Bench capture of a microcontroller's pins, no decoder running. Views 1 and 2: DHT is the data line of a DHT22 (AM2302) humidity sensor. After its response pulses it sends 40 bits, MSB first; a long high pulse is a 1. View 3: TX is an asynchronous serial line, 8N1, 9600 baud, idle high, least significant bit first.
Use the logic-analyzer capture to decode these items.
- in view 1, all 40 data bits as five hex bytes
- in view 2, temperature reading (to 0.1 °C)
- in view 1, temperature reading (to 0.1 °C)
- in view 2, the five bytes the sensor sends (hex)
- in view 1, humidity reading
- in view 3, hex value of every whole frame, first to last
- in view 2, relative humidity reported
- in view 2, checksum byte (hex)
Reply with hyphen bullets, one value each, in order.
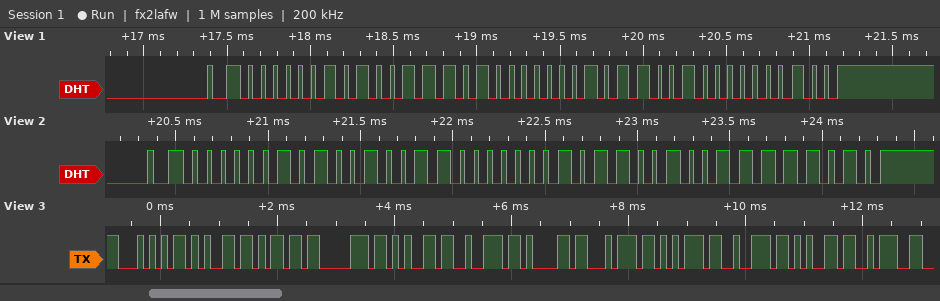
- 02 9D 01 64 04
- 35.6 °C
- 35.6 °C
- 02 93 01 64 FA
- 66.9 %
- 54 65 6D 70 65 72 61 74 75 72 65 3A
- 65.9 %
- 0xFA
